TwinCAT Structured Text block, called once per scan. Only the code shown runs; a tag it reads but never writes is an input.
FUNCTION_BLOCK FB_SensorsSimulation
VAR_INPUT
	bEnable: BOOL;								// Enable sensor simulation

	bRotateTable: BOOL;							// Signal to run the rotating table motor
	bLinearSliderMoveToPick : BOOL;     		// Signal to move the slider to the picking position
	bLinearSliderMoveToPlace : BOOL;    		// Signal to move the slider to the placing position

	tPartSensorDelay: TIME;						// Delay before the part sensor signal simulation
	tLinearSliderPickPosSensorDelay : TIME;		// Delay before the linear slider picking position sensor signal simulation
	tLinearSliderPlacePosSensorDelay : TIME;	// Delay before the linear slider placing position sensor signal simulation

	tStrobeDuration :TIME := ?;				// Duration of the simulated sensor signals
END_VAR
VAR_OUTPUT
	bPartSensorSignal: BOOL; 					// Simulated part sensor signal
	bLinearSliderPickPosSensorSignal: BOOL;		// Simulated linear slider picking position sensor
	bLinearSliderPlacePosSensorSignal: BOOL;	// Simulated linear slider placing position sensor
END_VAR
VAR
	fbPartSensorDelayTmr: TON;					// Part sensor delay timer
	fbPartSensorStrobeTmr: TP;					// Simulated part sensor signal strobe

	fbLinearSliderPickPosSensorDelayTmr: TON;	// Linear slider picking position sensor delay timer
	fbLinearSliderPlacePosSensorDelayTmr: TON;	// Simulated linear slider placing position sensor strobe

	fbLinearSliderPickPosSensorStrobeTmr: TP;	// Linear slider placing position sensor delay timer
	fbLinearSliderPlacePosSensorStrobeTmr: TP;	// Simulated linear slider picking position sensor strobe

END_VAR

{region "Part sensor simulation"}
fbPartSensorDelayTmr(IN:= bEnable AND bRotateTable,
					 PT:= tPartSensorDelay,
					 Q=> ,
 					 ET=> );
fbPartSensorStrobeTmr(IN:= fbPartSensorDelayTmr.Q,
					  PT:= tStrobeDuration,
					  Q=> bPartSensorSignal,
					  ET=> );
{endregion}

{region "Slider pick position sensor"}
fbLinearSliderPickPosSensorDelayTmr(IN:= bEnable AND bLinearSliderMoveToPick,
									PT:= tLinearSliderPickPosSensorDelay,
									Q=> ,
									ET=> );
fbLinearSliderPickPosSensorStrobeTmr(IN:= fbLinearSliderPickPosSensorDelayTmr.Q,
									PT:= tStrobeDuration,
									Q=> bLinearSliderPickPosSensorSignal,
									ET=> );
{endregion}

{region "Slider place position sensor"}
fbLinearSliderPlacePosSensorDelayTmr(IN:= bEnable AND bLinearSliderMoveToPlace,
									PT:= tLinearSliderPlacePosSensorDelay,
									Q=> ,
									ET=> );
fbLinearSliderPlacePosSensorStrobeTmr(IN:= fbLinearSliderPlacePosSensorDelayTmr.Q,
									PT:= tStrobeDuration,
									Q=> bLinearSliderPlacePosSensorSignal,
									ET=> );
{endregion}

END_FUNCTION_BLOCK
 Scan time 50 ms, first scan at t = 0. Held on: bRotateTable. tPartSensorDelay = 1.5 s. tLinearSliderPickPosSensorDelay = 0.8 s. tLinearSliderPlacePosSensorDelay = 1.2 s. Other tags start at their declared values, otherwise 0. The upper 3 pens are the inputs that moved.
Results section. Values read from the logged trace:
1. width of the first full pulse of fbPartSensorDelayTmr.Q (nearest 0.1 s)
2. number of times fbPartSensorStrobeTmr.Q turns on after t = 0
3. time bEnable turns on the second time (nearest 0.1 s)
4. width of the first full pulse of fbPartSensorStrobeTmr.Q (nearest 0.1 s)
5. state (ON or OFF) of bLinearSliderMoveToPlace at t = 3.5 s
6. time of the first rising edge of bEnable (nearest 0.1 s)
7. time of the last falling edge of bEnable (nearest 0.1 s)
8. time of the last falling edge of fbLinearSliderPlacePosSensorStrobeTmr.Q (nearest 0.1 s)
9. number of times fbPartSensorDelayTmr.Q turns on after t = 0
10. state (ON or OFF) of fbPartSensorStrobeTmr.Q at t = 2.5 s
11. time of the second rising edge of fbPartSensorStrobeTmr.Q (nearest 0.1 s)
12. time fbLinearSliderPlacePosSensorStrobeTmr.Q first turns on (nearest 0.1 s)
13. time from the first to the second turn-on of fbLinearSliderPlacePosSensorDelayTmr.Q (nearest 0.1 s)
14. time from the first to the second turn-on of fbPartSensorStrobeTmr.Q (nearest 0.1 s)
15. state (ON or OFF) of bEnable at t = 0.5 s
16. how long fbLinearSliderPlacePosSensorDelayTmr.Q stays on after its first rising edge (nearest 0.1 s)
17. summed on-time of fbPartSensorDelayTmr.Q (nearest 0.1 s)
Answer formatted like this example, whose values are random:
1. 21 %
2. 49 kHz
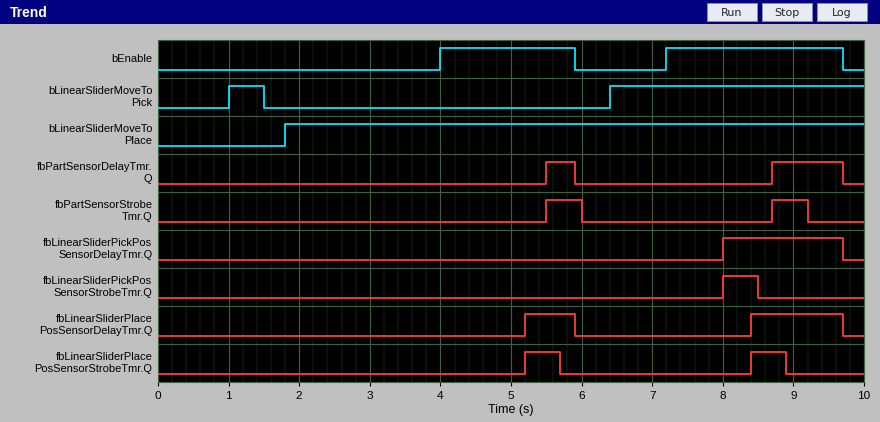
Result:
1. 0.4 s
2. 2
3. 7.2 s
4. 0.5 s
5. ON
6. 4.0 s
7. 9.7 s
8. 8.9 s
9. 2
10. OFF
11. 8.7 s
12. 5.2 s
13. 3.2 s
14. 3.2 s
15. OFF
16. 0.7 s
17. 1.4 s
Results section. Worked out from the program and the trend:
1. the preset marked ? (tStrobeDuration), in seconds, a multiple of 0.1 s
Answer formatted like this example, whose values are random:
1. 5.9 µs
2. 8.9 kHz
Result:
1. 0.5 s
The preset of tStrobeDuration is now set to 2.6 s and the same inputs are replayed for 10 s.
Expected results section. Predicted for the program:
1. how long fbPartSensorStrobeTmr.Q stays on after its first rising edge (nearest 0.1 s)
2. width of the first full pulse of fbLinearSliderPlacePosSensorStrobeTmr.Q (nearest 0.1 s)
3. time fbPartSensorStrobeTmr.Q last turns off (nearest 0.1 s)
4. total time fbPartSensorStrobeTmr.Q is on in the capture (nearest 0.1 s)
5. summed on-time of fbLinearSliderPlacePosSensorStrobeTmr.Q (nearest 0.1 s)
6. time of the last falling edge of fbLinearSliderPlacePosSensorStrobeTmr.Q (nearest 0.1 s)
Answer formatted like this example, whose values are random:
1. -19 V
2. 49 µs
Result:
1. 2.6 s
2. 2.6 s
3. 8.1 s
4. 3.9 s
5. 4.2 s
6. 7.8 s
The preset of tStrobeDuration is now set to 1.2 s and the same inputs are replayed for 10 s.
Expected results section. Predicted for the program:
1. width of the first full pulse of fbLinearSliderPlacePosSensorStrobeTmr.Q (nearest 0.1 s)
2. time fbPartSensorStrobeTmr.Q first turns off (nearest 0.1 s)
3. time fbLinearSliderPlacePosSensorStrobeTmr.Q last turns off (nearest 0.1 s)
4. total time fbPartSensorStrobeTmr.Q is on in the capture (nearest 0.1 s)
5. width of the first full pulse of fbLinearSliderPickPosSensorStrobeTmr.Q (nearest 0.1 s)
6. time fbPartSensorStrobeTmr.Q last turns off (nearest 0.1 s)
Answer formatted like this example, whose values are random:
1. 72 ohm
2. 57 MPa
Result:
1. 1.2 s
2. 6.7 s
3. 9.6 s
4. 2.4 s
5. 1.2 s
6. 9.9 s
